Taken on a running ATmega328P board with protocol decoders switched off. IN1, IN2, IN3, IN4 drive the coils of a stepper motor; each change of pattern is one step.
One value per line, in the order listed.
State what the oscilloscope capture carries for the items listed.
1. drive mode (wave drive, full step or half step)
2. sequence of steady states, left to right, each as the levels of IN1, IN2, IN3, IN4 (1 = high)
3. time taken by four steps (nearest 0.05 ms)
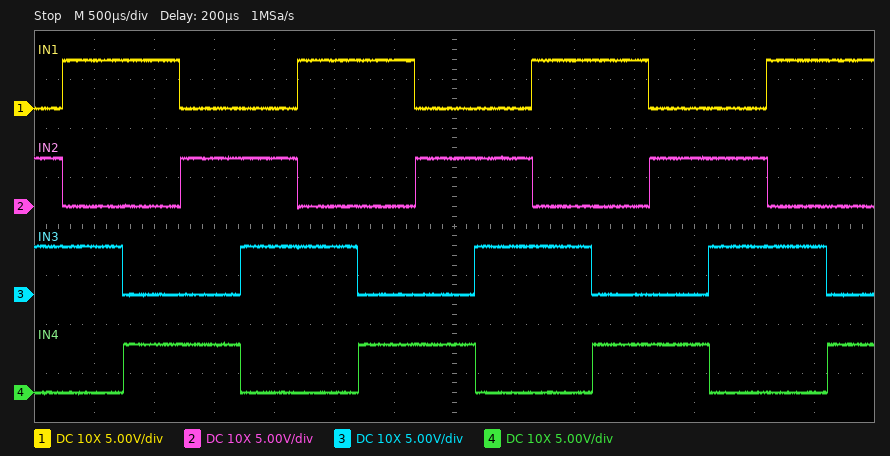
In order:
full step
0110 1010 1001 0101 0110 1010 1001 0101 0110 1010 1001 0101 0110 1010 1001
1.95 ms
